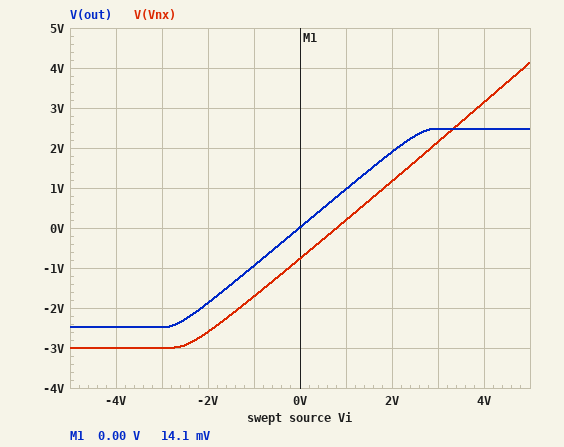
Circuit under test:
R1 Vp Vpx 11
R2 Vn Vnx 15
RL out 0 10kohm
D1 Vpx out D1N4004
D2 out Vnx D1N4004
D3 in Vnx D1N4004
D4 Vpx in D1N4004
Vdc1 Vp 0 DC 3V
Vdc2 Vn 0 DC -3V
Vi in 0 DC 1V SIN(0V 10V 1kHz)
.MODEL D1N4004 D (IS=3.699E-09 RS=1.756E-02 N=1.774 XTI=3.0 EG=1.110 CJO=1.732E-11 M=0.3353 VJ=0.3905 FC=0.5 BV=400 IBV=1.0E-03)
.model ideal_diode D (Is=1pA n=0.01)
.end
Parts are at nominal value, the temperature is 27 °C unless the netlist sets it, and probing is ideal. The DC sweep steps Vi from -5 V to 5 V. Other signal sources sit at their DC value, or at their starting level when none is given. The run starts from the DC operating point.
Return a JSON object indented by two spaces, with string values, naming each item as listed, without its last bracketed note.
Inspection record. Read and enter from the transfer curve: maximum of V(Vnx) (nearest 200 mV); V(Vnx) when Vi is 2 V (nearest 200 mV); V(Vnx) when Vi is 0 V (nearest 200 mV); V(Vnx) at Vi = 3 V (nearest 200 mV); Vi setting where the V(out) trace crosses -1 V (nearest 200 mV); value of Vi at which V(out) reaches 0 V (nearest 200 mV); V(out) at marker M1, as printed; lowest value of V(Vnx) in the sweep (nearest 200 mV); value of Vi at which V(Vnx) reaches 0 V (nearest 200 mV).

{
  "maximum of V(Vnx)": "4.2 V",
  "V(Vnx) when Vi is 2 V": "1.2 V",
  "V(Vnx) when Vi is 0 V": "-800 mV",
  "V(Vnx) at Vi = 3 V": "2.2 V",
  "Vi setting where the V(out) trace crosses -1 V": "-1.0 V",
  "value of Vi at which V(out) reaches 0 V": "0 V",
  "V(out) at marker M1, as printed": "14.1 mV",
  "lowest value of V(Vnx) in the sweep": "-3.0 V",
  "value of Vi at which V(Vnx) reaches 0 V": "800 mV"
}
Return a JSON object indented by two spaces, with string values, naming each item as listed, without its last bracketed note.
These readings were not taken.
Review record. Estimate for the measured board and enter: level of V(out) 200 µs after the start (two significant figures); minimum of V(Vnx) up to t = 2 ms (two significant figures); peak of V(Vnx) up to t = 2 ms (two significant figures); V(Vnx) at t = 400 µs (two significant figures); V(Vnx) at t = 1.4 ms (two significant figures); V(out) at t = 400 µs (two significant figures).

{
  "level of V(out) 200 µs after the start": "2.5 V",
  "minimum of V(Vnx) up to t = 2 ms": "-3.0 V",
  "peak of V(Vnx) up to t = 2 ms": "9.1 V",
  "V(Vnx) at t = 400 µs": "5.0 V",
  "V(Vnx) at t = 1.4 ms": "5.0 V",
  "V(out) at t = 400 µs": "2.5 V"
}
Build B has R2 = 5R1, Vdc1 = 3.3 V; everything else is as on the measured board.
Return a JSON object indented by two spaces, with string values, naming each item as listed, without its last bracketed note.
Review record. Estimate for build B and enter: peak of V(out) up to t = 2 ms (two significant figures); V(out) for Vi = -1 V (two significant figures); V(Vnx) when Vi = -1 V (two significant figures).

{
  "peak of V(out) up to t = 2 ms": "2.8 V",
  "V(out) for Vi = -1 V": "-990 mV",
  "V(Vnx) when Vi = -1 V": "-1.8 V"
}
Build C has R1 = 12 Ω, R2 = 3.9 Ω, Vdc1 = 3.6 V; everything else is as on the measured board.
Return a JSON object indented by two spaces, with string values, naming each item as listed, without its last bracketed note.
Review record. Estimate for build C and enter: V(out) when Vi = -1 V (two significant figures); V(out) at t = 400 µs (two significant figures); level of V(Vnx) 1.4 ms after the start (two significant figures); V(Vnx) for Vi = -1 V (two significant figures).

{
  "V(out) when Vi = -1 V": "-1.0 V",
  "V(out) at t = 400 µs": "3.1 V",
  "level of V(Vnx) 1.4 ms after the start": "4.9 V",
  "V(Vnx) for Vi = -1 V": "-1.8 V"
}
